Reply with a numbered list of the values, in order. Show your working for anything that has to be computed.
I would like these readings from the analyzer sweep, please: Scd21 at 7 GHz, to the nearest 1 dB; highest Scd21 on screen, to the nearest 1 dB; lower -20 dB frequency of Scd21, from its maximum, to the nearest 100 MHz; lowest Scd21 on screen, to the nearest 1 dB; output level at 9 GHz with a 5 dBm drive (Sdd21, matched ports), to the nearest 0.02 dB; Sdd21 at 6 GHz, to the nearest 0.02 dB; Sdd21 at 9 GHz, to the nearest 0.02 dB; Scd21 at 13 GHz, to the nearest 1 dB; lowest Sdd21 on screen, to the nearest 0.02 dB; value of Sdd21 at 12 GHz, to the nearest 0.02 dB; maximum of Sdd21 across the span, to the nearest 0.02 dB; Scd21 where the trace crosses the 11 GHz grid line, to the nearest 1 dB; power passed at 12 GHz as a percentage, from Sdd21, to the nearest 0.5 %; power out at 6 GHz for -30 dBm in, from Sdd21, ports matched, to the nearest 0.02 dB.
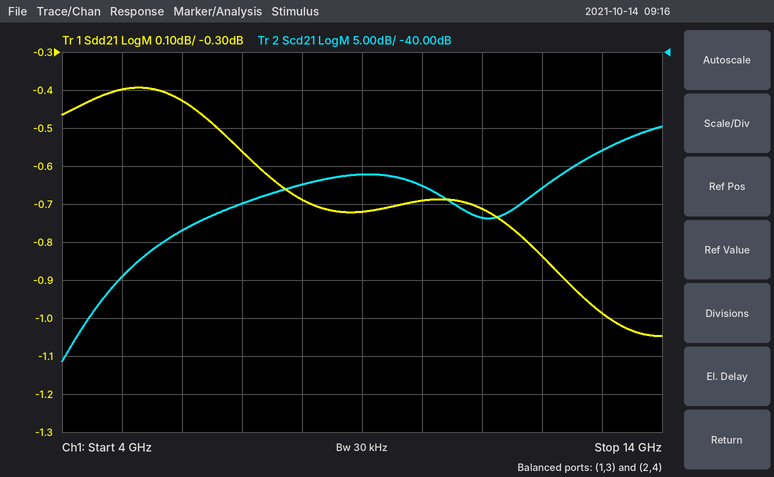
1. -60 dB
2. -50 dB
3. 5.0 GHz
4. -81 dB
5. 5 dBm + (-0.72 dB) = 4.28 dBm
6. -0.42 dB
7. -0.72 dB
8. -53 dB
9. -1.04 dB
10. -0.84 dB
11. -0.40 dB
12. -62 dB
13. 10^(-0.84/10) ≈ 82.4 %, so 82.5 % to the nearest 0.5 %
14. -30 dBm + (-0.42 dB) = -30.42 dBm
